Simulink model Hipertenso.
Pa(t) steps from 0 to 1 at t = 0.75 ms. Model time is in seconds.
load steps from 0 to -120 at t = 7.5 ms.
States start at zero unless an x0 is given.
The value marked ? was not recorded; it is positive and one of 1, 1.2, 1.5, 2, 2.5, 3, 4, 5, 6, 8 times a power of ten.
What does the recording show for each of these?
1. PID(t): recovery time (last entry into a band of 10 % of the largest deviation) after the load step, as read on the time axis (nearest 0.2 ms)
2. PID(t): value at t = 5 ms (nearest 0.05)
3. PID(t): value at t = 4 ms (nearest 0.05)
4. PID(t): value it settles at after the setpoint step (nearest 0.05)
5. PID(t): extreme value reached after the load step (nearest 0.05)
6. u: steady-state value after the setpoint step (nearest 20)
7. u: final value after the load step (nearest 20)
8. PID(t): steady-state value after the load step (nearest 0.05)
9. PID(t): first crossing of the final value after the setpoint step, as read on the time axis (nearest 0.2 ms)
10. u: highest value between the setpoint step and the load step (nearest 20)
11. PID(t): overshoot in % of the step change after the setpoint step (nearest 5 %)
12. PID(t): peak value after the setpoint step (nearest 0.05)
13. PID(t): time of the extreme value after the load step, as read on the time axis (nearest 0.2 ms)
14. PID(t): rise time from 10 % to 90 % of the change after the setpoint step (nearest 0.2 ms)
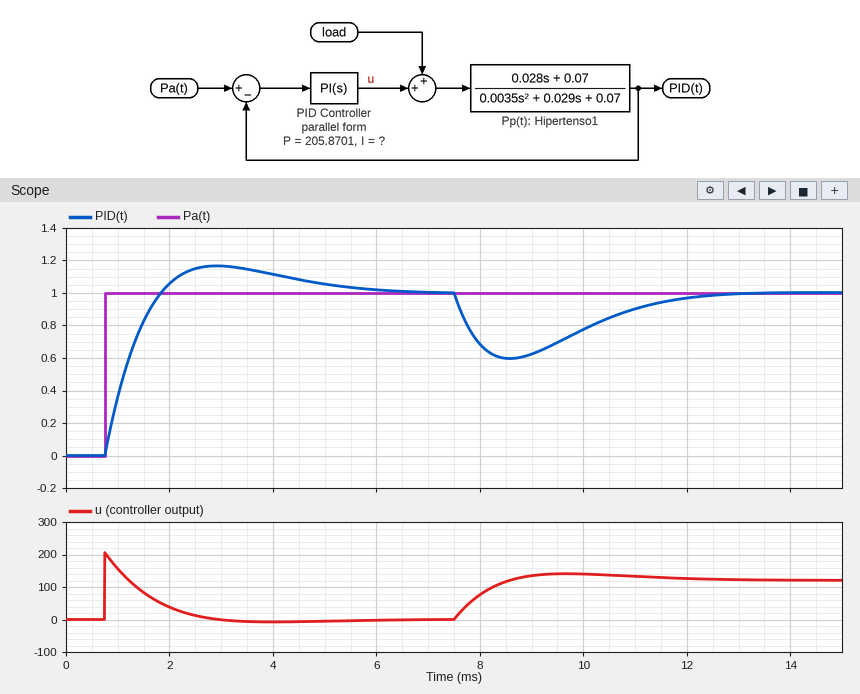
11.8 ms
1.05
1.10
1.00
0.60
0
120
1.00
1.8 ms
200
15 %
1.15
8.6 ms
0.8 ms
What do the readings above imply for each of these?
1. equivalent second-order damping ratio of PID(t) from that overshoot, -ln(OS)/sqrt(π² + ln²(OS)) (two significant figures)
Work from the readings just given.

0.52
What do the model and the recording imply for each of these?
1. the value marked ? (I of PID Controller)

120000
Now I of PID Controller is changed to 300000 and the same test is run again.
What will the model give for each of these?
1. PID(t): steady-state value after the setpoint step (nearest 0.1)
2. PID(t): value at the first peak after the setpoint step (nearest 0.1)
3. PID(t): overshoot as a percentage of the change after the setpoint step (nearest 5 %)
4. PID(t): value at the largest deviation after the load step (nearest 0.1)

1.0
1.3
30 %
0.7
